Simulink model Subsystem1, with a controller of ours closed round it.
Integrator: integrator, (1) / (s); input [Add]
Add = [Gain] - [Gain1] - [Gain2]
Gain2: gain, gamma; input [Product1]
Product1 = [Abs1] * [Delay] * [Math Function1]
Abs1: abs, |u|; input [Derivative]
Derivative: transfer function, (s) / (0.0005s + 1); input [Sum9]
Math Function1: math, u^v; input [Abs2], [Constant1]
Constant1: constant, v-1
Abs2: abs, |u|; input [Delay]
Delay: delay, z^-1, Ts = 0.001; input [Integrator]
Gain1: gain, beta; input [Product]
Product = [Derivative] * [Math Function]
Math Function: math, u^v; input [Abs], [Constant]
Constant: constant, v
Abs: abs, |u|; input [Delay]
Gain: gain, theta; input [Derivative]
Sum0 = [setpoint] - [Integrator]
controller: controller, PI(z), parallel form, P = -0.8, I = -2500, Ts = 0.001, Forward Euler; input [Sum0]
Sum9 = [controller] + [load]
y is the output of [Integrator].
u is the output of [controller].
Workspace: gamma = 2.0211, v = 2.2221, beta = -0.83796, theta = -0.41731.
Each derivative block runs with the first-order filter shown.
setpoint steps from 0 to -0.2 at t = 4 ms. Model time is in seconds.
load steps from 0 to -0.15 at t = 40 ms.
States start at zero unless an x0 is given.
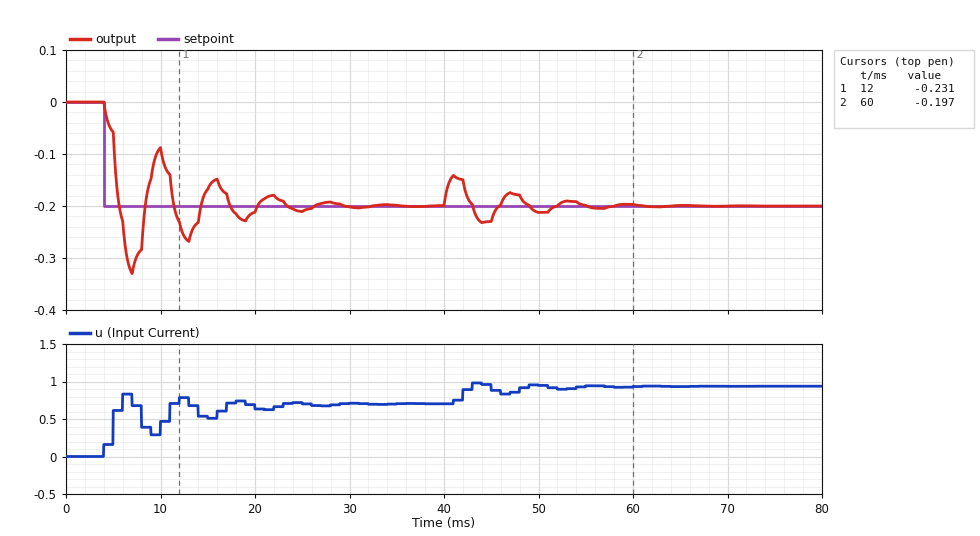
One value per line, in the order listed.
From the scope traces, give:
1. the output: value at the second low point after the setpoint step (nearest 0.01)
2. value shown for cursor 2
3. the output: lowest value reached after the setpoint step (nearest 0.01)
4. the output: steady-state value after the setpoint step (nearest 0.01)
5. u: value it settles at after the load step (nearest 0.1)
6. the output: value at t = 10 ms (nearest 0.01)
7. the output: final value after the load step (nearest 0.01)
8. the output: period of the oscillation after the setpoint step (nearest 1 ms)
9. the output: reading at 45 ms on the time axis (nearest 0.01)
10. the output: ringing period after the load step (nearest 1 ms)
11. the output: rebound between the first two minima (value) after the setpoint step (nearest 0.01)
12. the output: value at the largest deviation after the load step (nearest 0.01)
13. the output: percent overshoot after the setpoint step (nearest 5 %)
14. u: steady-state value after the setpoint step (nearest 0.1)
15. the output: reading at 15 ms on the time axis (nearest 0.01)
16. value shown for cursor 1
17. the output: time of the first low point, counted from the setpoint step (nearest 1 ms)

-0.27
-0.197
-0.33
-0.20
0.9
-0.09
-0.20
6 ms
-0.23
6 ms
-0.09
-0.14
65 %
0.7
-0.17
-0.231
3 ms
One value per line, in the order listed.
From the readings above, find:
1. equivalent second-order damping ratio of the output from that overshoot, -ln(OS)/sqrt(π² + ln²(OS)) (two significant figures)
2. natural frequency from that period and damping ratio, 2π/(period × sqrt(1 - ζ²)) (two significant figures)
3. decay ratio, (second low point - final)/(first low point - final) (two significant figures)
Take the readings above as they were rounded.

0.14
1.1 rad/ms
0.54
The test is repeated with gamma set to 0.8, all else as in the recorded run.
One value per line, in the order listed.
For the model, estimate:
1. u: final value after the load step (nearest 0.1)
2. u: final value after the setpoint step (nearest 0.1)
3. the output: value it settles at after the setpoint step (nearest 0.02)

0.7
0.5
-0.20
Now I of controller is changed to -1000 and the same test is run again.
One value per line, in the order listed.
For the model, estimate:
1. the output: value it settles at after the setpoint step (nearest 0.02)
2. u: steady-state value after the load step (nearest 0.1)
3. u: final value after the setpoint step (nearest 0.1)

-0.20
0.7
0.5
